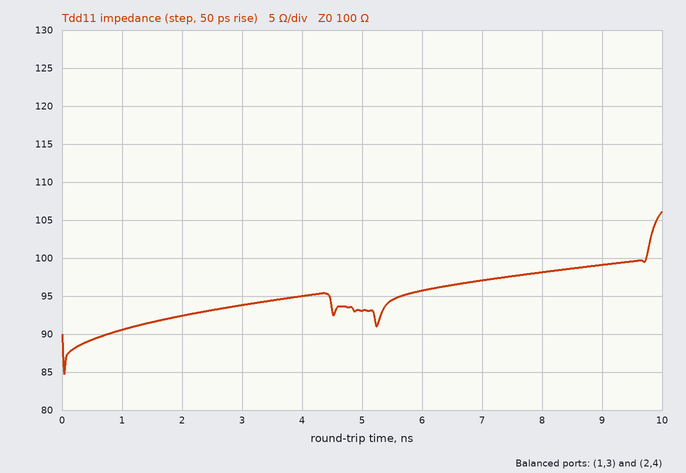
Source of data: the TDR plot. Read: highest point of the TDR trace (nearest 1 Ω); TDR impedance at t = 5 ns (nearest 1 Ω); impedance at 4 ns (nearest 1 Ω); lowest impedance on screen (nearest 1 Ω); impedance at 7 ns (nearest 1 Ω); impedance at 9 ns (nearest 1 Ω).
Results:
106 Ω
93 Ω
95 Ω
85 Ω
97 Ω
99 Ω
